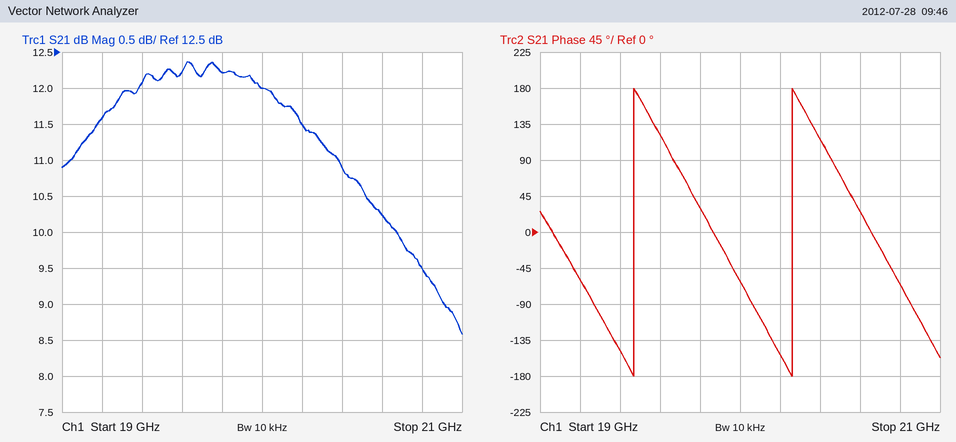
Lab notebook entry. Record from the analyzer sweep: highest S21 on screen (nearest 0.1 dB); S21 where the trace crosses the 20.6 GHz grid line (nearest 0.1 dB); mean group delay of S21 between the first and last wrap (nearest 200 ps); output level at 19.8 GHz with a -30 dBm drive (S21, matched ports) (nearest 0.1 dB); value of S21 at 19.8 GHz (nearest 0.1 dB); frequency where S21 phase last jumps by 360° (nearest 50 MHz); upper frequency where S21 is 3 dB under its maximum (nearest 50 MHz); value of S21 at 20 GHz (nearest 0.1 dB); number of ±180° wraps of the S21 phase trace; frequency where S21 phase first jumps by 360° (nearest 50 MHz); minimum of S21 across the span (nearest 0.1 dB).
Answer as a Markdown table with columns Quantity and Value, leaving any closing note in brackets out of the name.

| Quantity | Value |
|---|---|
| highest S21 on screen | 12.4 dB |
| S21 where the trace crosses the 20.6 GHz grid line | 10.2 dB |
| mean group delay of S21 between the first and last wrap | 1.2 ns |
| output level at 19.8 GHz with a -30 dBm drive (S21, matched ports) | -17.8 dBm |
| value of S21 at 19.8 GHz | 12.2 dB |
| frequency where S21 phase last jumps by 360° | 20.25 GHz |
| upper frequency where S21 is 3 dB under its maximum | 20.85 GHz |
| value of S21 at 20 GHz | 12.0 dB |
| number of ±180° wraps of the S21 phase trace | 2 |
| frequency where S21 phase first jumps by 360° | 19.45 GHz |
| minimum of S21 across the span | 8.6 dB |
